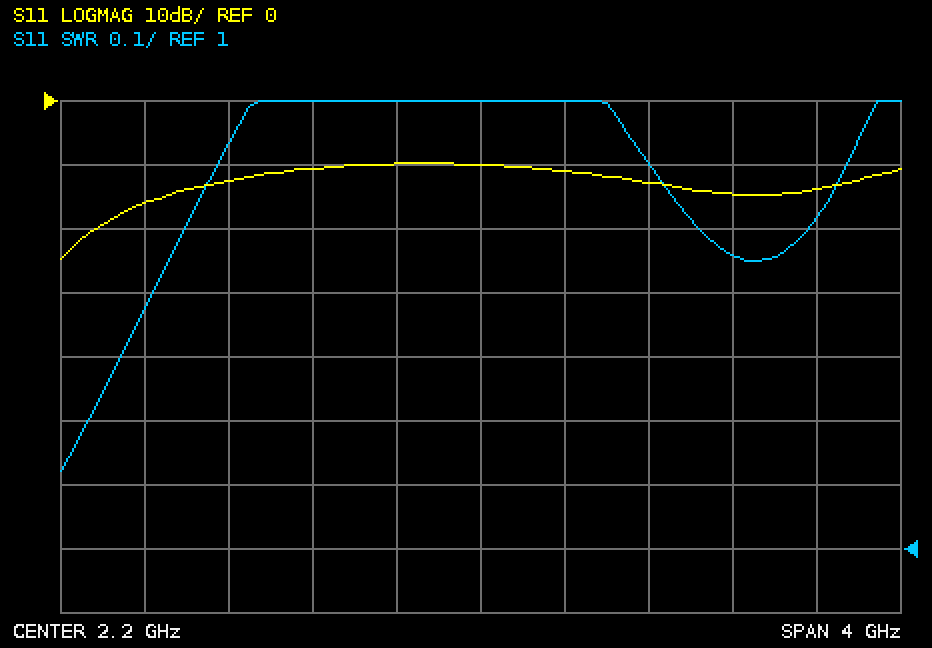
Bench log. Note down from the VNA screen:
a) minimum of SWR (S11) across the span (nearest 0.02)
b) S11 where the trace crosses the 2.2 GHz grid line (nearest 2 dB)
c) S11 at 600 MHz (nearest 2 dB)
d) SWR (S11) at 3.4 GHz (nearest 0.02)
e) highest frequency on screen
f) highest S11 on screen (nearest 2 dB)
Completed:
1.12
-10 dB
-16 dB
1.46
4.2 GHz
-10 dB
